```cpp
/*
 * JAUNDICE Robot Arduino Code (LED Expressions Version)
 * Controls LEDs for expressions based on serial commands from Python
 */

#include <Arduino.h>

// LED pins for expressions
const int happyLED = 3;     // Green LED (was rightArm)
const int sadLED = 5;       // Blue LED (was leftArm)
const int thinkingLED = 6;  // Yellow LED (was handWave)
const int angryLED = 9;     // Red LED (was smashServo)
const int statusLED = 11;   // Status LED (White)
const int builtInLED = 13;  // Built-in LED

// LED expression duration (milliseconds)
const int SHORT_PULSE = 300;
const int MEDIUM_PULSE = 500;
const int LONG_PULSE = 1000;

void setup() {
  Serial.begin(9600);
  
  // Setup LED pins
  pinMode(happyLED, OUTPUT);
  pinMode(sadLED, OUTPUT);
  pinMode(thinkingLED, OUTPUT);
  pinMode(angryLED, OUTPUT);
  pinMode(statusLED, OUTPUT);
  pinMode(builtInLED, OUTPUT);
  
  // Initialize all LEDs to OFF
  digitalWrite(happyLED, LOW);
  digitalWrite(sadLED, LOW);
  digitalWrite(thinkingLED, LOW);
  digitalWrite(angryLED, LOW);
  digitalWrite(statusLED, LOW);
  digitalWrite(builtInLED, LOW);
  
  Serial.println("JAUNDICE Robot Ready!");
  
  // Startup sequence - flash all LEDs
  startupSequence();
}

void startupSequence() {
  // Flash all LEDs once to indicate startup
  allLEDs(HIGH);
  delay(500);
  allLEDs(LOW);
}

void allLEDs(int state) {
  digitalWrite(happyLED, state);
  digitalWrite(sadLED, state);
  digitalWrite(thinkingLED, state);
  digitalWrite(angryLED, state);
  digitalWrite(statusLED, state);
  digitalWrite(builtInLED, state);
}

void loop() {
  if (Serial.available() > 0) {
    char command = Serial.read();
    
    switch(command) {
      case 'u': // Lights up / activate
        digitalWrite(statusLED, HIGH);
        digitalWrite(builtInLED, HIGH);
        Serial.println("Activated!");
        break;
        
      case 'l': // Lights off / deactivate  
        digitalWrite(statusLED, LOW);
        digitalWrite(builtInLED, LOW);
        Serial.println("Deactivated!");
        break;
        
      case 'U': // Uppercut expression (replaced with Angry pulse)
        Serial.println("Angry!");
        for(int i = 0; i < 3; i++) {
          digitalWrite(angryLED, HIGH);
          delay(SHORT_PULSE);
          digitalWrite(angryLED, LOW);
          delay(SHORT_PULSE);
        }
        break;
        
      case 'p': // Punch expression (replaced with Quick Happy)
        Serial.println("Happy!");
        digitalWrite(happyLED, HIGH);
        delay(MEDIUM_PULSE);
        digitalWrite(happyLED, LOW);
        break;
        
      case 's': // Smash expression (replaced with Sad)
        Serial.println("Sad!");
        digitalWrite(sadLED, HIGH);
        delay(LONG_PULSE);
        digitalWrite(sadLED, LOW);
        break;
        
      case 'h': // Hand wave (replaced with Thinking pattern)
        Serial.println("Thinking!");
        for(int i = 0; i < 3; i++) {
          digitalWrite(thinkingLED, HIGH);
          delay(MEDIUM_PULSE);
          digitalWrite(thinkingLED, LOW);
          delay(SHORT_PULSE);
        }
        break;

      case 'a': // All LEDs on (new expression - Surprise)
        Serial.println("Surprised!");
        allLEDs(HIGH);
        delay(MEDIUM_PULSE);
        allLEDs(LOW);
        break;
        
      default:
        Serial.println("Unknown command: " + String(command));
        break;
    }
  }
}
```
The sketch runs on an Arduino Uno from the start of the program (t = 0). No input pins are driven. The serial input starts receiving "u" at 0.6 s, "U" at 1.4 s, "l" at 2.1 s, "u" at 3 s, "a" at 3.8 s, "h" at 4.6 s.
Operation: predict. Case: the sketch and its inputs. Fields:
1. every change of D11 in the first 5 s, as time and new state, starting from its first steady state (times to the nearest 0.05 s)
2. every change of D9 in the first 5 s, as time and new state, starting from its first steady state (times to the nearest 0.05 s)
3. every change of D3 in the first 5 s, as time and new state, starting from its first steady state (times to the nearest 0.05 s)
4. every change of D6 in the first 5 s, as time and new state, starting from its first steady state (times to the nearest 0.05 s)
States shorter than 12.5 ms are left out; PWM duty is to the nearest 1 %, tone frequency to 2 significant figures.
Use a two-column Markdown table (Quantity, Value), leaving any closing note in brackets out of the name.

| Quantity | Value |
|---|---|
| every change of D11 in the first 5 s, as time and new state, starting from its first steady state | 0 s high; 0.5 s low; 0.6 s high; 4.3 s low |
| every change of D9 in the first 5 s, as time and new state, starting from its first steady state | 0 s high; 0.5 s low; 1.4 s high; 1.7 s low; 2 s high; 2.3 s low; 2.6 s high; 2.9 s low; 3.8 s high; 4.3 s low |
| every change of D3 in the first 5 s, as time and new state, starting from its first steady state | 0 s high; 0.5 s low; 3.8 s high; 4.3 s low |
| every change of D6 in the first 5 s, as time and new state, starting from its first steady state | 0 s high; 0.5 s low; 3.8 s high; 4.3 s low; 4.6 s high |
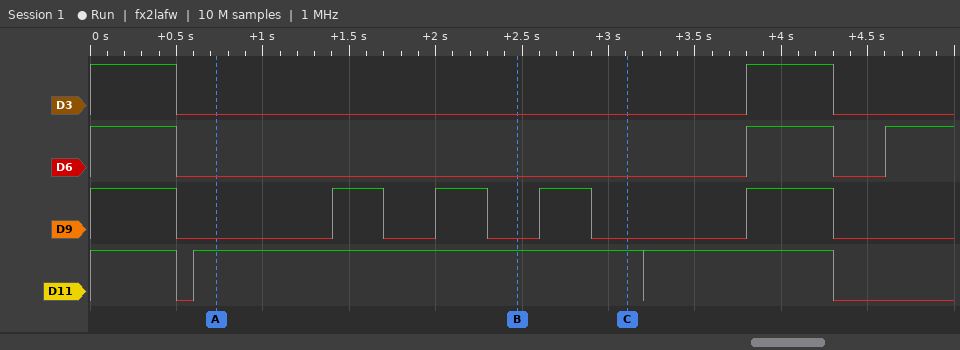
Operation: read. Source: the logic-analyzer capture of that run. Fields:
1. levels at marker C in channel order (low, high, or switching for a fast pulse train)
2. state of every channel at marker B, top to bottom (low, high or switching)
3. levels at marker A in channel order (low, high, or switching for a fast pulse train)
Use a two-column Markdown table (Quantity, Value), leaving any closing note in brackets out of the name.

| Quantity | Value |
|---|---|
| levels at marker C in channel order | D3 low, D6 low, D9 low, D11 high |
| state of every channel at marker B, top to bottom | D3 low, D6 low, D9 low, D11 high |
| levels at marker A in channel order | D3 low, D6 low, D9 low, D11 high |
